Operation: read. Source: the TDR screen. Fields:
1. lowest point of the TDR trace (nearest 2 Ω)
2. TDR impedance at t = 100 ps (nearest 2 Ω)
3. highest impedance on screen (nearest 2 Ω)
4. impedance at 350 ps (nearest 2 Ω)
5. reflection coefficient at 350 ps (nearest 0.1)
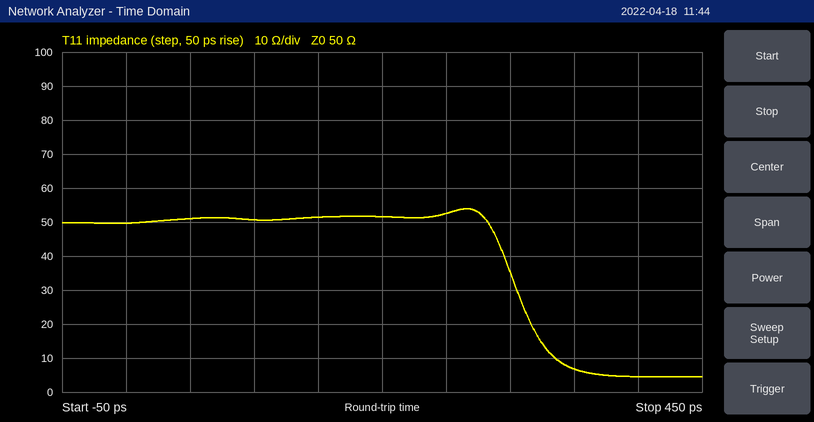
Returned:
4 Ω
50 Ω
54 Ω
6 Ω
-0.8
